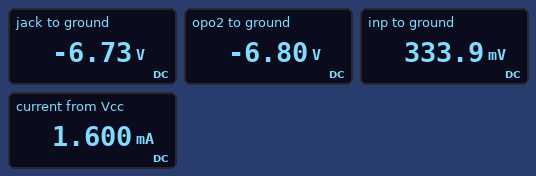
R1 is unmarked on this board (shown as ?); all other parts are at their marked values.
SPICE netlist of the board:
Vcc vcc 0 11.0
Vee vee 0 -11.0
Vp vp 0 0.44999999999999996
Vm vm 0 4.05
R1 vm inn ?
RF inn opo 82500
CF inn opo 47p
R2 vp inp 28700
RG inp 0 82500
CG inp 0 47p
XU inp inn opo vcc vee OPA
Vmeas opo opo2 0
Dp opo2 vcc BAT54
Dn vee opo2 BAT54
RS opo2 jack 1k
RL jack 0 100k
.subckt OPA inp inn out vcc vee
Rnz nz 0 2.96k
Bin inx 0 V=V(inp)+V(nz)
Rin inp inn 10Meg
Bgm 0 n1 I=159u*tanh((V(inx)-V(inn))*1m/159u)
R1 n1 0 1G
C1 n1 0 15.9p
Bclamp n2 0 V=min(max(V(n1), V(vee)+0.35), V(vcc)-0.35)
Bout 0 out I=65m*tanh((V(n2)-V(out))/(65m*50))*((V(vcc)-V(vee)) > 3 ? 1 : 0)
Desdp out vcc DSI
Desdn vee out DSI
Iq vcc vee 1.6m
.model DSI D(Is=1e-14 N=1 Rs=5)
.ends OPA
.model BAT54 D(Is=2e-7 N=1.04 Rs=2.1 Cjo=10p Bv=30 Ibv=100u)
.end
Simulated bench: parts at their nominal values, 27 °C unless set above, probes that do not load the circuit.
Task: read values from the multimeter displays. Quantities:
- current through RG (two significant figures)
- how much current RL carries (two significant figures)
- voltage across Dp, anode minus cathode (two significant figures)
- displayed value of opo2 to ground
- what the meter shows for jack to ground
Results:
4.0 µA
67 µA
-18 V
-6.80 V
-6.73 V
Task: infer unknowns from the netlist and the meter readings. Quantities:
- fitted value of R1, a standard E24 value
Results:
43 kΩ
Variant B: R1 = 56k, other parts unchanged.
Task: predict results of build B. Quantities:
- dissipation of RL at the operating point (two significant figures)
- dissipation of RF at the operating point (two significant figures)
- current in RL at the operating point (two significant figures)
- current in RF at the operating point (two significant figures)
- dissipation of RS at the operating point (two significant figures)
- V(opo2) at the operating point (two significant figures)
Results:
260 µW
360 µW
51 µA
66 µA
2.6 µW
-5.1 V
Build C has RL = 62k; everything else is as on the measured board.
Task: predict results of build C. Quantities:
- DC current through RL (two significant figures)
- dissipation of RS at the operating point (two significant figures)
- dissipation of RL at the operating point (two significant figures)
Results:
110 µA
12 µW
720 µW
